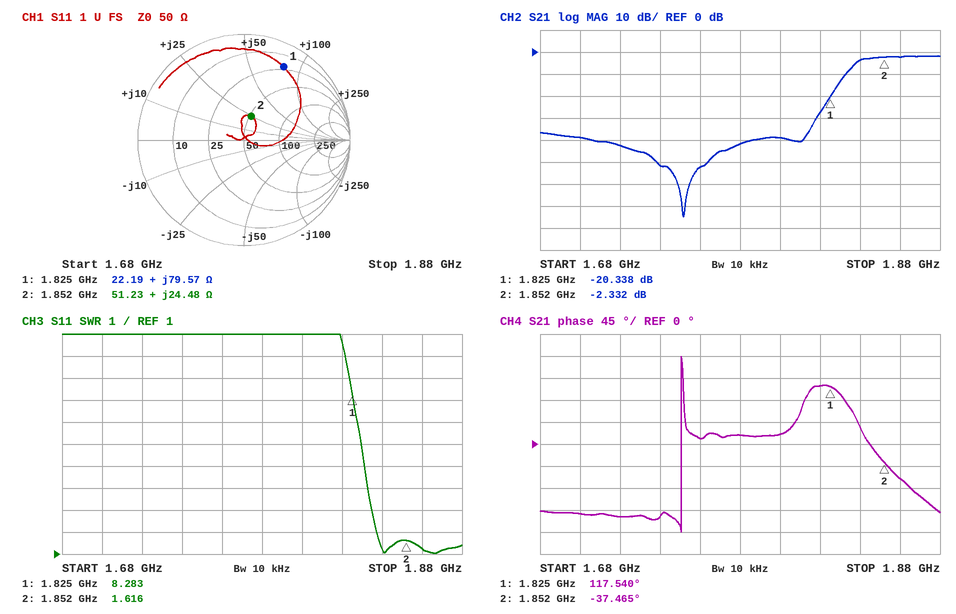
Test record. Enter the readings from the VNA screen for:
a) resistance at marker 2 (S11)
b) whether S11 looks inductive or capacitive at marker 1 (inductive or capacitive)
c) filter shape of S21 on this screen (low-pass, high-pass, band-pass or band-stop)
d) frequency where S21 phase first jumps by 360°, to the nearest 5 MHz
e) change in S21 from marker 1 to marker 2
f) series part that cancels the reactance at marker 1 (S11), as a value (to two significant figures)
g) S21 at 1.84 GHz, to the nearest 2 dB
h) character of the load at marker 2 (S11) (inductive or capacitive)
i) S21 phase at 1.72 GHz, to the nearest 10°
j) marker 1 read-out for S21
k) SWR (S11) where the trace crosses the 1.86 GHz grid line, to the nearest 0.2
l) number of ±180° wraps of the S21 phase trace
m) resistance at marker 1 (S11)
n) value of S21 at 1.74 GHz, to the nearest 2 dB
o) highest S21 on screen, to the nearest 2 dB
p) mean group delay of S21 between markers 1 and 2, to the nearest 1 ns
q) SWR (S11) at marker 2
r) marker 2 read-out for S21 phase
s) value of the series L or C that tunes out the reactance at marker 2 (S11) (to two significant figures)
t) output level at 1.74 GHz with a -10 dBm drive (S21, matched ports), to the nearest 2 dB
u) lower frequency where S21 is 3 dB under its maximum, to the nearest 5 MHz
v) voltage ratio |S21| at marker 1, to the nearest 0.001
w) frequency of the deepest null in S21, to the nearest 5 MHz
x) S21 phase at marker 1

51.23 Ω
inductive
high-pass
1.750 GHz
18.006 dB
1.1 pF
-4 dB
inductive
-150°
-20.338 dB
1.2
1
22.19 Ω
-52 dB
-2 dB
16 ns
1.616
-37.465°
3.5 pF
-62 dBm
1.840 GHz
0.096
1.750 GHz
117.540°
